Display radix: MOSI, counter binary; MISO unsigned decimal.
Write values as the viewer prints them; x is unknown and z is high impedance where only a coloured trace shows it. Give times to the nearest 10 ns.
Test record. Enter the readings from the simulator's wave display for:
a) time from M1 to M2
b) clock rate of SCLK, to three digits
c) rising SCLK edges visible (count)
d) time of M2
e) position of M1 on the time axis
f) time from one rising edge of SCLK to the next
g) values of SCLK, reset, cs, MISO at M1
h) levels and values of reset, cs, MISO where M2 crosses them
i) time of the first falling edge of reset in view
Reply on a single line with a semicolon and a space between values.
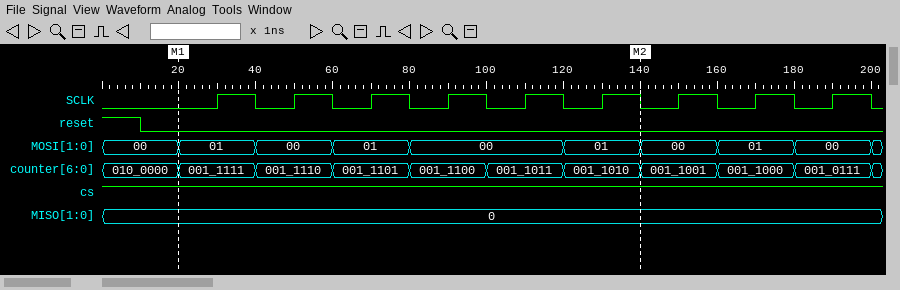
120 ns; 50.0 MHz; 9; 140 ns; 20 ns; 20 ns; SCLK=0, reset=0, cs=1, MISO=0; reset=0, cs=1, MISO=0; 10 ns
